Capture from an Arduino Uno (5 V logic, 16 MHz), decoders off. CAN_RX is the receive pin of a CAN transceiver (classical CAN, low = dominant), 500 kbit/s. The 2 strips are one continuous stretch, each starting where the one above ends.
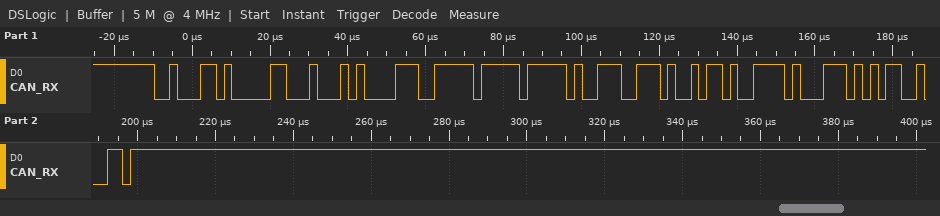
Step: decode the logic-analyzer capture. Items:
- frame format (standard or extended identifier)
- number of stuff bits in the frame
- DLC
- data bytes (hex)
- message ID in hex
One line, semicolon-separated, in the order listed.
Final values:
standard; 4; 8; 8A 1C FF FF 39 D2 D3 D1; 0x234
